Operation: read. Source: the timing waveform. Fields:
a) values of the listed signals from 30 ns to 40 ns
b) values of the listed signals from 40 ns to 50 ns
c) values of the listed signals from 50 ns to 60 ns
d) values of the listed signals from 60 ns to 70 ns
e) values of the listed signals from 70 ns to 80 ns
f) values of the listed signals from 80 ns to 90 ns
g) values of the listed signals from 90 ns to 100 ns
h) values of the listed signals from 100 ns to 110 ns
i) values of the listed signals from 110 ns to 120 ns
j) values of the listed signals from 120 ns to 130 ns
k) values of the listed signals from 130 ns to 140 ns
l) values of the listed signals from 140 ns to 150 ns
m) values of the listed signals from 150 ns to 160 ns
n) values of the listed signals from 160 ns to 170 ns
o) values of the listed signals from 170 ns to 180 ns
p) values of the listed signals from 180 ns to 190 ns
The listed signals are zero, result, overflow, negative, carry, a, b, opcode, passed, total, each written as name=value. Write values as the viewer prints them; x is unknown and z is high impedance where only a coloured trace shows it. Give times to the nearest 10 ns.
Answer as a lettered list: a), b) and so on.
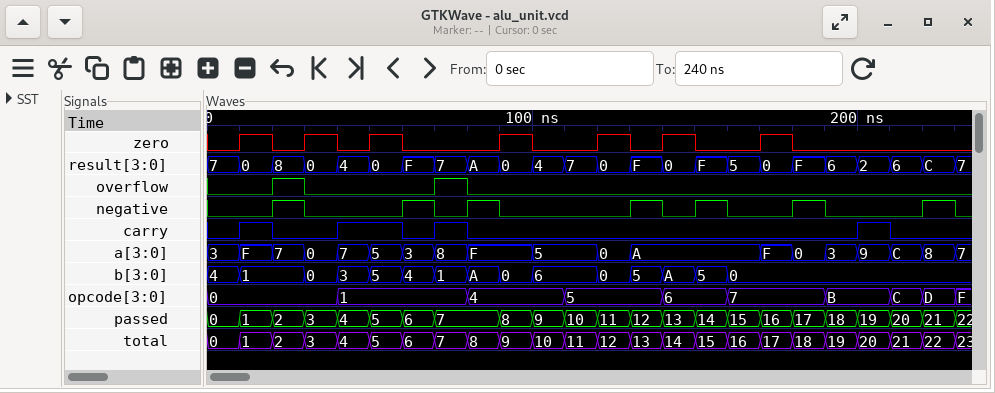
a) zero=1, result=0, overflow=0, negative=0, carry=0, a=0, b=0, opcode=0, passed=3, total=3
b) zero=0, result=4, overflow=0, negative=0, carry=1, a=7, b=3, opcode=1, passed=4, total=4
c) zero=1, result=0, overflow=0, negative=0, carry=1, a=5, b=5, opcode=1, passed=5, total=5
d) zero=0, result=F, overflow=0, negative=1, carry=0, a=3, b=4, opcode=1, passed=6, total=6
e) zero=0, result=7, overflow=1, negative=0, carry=1, a=8, b=1, opcode=1, passed=7, total=7
f) zero=0, result=A, overflow=0, negative=1, carry=0, a=F, b=A, opcode=4, passed=7, total=8
g) zero=1, result=0, overflow=0, negative=0, carry=0, a=F, b=0, opcode=4, passed=8, total=9
h) zero=0, result=4, overflow=0, negative=0, carry=0, a=5, b=6, opcode=4, passed=9, total=10
i) zero=0, result=7, overflow=0, negative=0, carry=0, a=5, b=6, opcode=5, passed=10, total=11
j) zero=1, result=0, overflow=0, negative=0, carry=0, a=0, b=0, opcode=5, passed=11, total=12
k) zero=0, result=F, overflow=0, negative=1, carry=0, a=A, b=5, opcode=5, passed=12, total=13
l) zero=1, result=0, overflow=0, negative=0, carry=0, a=A, b=A, opcode=6, passed=13, total=14
m) zero=0, result=F, overflow=0, negative=1, carry=0, a=A, b=5, opcode=6, passed=14, total=15
n) zero=0, result=5, overflow=0, negative=0, carry=0, a=A, b=0, opcode=7, passed=15, total=16
o) zero=1, result=0, overflow=0, negative=0, carry=0, a=F, b=0, opcode=7, passed=16, total=17
p) zero=0, result=F, overflow=0, negative=1, carry=0, a=0, b=0, opcode=7, passed=17, total=18
